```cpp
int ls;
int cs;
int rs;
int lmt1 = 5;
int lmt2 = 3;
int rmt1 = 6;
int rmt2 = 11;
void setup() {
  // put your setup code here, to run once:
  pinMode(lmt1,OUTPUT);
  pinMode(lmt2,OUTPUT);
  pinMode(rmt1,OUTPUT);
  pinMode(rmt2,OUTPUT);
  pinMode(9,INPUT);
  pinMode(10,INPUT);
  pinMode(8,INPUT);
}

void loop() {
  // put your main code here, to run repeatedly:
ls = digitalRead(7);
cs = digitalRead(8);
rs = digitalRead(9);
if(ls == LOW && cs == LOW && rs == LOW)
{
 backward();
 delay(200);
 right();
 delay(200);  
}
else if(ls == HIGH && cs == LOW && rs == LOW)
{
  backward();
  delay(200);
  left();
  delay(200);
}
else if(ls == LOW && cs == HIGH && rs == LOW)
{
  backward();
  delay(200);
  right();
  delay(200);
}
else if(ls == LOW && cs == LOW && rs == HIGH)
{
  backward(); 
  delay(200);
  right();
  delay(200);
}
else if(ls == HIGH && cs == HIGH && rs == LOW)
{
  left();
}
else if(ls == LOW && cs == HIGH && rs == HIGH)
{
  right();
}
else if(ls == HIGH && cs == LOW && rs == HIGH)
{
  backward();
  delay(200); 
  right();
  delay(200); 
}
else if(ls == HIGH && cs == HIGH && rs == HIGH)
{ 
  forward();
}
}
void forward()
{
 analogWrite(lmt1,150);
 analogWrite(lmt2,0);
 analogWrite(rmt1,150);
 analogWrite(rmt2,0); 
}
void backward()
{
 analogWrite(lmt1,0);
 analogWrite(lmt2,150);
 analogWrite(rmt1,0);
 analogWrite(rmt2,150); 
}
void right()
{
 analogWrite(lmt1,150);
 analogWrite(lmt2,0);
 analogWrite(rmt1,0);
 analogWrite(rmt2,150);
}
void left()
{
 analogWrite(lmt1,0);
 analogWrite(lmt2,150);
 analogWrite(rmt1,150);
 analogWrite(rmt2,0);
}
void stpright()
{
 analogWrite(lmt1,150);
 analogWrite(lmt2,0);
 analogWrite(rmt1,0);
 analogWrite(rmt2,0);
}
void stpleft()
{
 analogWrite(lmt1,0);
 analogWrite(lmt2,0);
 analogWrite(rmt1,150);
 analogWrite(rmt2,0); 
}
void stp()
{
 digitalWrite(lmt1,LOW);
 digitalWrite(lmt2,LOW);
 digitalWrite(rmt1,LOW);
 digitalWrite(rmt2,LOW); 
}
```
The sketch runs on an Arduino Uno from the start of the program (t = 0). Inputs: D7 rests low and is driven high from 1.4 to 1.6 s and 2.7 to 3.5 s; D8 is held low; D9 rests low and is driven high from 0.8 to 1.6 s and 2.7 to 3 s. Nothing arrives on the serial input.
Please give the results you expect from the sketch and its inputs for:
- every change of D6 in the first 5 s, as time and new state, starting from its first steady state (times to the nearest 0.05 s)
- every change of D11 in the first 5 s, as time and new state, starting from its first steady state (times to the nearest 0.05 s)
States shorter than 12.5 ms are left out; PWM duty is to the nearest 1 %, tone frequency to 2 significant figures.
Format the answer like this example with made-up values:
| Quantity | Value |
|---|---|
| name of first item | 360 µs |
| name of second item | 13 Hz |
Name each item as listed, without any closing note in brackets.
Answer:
| Quantity | Value |
|---|---|
| every change of D6 in the first 5 s, as time and new state, starting from its first steady state | 0 s low; 3.4 s PWM 59 %; 3.6 s low |
| every change of D11 in the first 5 s, as time and new state, starting from its first steady state | 0 s PWM 59 %; 3.4 s low; 3.6 s PWM 59 % |
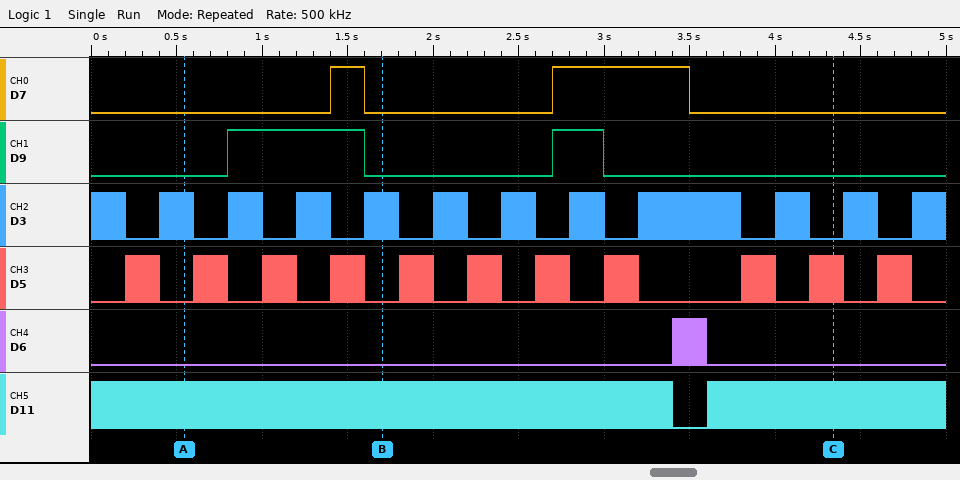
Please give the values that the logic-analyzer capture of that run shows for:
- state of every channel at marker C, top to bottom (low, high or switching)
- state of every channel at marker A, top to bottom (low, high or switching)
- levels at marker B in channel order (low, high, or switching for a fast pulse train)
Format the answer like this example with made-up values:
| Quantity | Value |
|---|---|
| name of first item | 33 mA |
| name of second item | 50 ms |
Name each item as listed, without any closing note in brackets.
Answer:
| Quantity | Value |
|---|---|
| state of every channel at marker C, top to bottom | D7 low, D9 low, D3 low, D5 switching, D6 low, D11 switching |
| state of every channel at marker A, top to bottom | D7 low, D9 low, D3 switching, D5 low, D6 low, D11 switching |
| levels at marker B in channel order | D7 low, D9 low, D3 switching, D5 low, D6 low, D11 switching |
